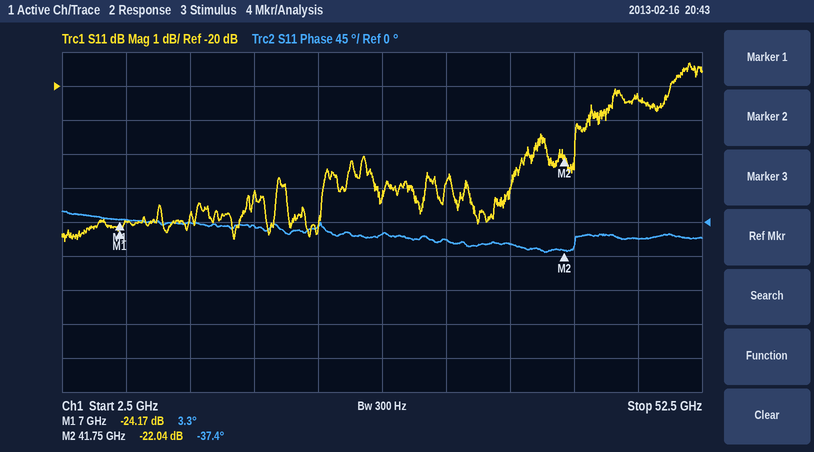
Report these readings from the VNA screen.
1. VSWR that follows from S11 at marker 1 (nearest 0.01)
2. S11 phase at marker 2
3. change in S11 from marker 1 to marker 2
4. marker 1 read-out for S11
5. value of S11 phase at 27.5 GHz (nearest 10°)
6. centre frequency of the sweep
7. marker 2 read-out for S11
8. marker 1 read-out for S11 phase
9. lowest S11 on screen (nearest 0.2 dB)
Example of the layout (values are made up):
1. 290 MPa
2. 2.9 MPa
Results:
1. 1.13
2. -37.4°
3. 2.13 dB
4. -24.17 dB
5. -20°
6. 27.5 GHz
7. -22.04 dB
8. 3.3°
9. -24.6 dB
